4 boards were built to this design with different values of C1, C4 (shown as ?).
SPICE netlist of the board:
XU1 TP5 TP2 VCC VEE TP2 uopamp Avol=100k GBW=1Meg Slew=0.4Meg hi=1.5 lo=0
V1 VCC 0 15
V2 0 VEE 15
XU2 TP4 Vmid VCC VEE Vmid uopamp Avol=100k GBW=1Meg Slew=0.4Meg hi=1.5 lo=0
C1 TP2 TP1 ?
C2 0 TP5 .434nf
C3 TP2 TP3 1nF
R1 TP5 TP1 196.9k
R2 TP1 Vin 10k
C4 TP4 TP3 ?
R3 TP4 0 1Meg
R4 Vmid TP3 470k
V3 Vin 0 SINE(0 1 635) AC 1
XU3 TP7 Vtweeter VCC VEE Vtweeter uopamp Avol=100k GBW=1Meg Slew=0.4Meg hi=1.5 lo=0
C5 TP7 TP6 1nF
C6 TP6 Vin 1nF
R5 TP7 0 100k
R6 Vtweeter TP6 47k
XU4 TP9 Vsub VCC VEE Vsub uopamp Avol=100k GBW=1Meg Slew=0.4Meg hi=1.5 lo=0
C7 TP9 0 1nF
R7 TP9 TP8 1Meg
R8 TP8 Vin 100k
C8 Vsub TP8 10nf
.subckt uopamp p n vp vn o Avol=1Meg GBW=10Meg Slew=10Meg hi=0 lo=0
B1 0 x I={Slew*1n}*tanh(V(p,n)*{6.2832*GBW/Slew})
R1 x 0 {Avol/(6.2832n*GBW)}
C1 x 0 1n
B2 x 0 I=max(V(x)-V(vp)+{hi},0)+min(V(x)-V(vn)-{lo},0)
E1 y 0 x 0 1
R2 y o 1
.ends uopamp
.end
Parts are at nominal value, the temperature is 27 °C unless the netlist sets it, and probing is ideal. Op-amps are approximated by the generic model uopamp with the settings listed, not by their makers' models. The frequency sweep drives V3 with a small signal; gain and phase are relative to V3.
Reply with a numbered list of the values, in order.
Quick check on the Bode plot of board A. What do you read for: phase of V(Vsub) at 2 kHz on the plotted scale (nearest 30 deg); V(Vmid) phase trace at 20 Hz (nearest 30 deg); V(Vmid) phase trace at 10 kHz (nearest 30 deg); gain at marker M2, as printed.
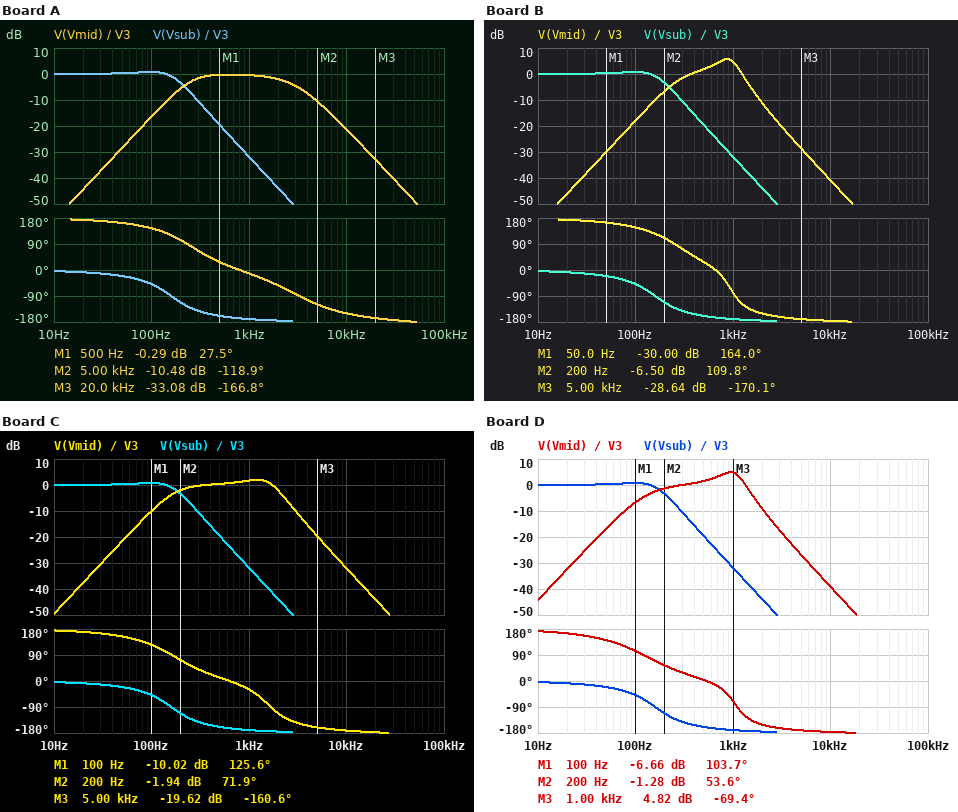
1. -180 deg
2. 180 deg
3. -150 deg
4. -10.48 dB
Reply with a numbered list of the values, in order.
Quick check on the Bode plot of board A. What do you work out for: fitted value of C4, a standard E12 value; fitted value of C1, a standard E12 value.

1. 820 pF
2. 3.3 nF
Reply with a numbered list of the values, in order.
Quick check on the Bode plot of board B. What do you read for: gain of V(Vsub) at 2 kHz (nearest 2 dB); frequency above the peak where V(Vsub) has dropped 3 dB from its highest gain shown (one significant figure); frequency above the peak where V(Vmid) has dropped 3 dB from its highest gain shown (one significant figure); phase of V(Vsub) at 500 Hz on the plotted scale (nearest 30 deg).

1. -44 dB
2. 200 Hz
3. 1 kHz
4. -150 deg
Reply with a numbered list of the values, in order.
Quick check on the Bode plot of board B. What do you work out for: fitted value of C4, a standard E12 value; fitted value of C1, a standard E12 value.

1. 680 pF
2. 33 nF
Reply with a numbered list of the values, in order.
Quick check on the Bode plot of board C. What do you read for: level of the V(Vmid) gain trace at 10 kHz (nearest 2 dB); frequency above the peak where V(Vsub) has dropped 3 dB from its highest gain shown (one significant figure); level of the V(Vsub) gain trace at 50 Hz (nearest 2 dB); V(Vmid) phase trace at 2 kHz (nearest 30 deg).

1. -32 dB
2. 200 Hz
3. 0 dB
4. -120 deg
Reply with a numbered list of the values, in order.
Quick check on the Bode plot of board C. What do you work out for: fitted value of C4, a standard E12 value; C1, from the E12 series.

1. 1.8 nF
2. 12 nF
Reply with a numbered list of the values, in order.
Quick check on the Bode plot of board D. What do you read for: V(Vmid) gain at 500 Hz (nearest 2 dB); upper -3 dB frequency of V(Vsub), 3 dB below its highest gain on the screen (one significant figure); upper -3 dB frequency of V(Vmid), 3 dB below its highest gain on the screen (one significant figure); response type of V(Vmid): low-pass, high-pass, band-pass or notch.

1. 2 dB
2. 200 Hz
3. 1 kHz
4. band-pass
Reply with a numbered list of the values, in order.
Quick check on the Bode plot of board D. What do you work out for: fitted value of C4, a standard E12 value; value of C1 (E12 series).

1. 3.3 nF
2. 27 nF
